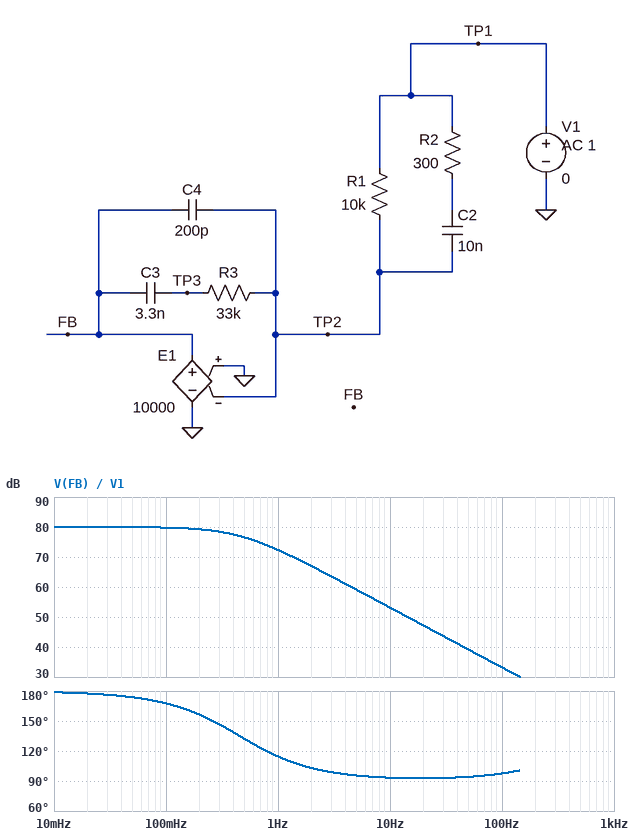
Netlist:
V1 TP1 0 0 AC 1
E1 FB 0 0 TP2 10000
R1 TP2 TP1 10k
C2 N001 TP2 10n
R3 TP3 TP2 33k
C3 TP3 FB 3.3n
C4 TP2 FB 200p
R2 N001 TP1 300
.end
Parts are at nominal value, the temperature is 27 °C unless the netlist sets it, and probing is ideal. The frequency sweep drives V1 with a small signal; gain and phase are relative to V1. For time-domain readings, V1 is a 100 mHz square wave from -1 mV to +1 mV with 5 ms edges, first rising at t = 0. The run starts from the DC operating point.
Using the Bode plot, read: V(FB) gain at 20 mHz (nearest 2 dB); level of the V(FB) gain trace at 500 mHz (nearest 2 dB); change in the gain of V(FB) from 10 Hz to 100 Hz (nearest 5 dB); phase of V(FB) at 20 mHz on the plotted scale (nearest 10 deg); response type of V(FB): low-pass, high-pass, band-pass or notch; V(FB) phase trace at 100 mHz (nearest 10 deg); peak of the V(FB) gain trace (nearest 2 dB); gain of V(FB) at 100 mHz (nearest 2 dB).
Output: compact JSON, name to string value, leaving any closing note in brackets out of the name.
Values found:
{"V(FB) gain at 20 mHz": "80 dB", "level of the V(FB) gain trace at 500 mHz": "76 dB", "change in the gain of V(FB) from 10 Hz to 100 Hz": "-20 dB", "phase of V(FB) at 20 mHz on the plotted scale": "180 deg", "response type of V(FB): low-pass, high-pass, band-pass or notch": "low-pass", "V(FB) phase trace at 100 mHz": "170 deg", "peak of the V(FB) gain trace": "80 dB", "gain of V(FB) at 100 mHz": "80 dB"}
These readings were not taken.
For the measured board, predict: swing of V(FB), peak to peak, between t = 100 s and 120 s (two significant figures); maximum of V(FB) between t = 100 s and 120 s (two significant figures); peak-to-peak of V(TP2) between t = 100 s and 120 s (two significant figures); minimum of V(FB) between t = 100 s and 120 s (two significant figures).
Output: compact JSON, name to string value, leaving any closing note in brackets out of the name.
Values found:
{"swing of V(FB), peak to peak, between t = 100 s and 120 s": "20 V", "maximum of V(FB) between t = 100 s and 120 s": "10 V", "peak-to-peak of V(TP2) between t = 100 s and 120 s": "2.0 mV", "minimum of V(FB) between t = 100 s and 120 s": "-10 V"}
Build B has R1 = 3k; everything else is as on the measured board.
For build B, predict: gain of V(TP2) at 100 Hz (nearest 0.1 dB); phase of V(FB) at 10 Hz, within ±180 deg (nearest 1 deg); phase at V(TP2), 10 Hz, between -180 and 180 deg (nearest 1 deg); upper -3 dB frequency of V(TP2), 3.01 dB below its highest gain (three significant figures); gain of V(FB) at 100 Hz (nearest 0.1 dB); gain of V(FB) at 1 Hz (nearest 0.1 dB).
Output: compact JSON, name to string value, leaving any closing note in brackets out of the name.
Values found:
{"gain of V(TP2) at 100 Hz": "-36.4 dB", "phase of V(FB) at 10 Hz, within ±180 deg": "99 deg", "phase at V(TP2), 10 Hz, between -180 and 180 deg": "-81 deg", "upper -3 dB frequency of V(TP2), 3.01 dB below its highest gain": "1.51 Hz", "gain of V(FB) at 100 Hz": "43.6 dB", "gain of V(FB) at 1 Hz": "78.4 dB"}
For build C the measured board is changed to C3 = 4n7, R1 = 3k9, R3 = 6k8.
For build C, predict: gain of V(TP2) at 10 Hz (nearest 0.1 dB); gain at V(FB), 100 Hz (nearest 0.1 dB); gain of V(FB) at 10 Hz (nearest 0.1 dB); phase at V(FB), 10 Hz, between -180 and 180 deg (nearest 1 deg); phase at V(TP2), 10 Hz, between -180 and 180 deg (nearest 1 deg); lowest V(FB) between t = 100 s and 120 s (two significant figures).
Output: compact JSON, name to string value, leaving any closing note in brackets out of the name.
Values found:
{"gain of V(TP2) at 10 Hz": "-21.6 dB", "gain at V(FB), 100 Hz": "38.4 dB", "gain of V(FB) at 10 Hz": "58.4 dB", "phase at V(FB), 10 Hz, between -180 and 180 deg": "95 deg", "phase at V(TP2), 10 Hz, between -180 and 180 deg": "-85 deg", "lowest V(FB) between t = 100 s and 120 s": "-10 V"}
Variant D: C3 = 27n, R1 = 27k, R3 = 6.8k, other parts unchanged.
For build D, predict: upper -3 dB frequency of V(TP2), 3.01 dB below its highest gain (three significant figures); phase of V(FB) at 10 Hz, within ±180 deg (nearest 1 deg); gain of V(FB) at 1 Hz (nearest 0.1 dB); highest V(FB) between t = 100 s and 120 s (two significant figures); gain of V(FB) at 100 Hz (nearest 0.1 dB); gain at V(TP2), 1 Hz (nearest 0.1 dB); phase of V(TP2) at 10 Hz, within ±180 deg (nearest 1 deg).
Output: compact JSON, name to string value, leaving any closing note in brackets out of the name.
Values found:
{"upper -3 dB frequency of V(TP2), 3.01 dB below its highest gain": "21.7 mHz", "phase of V(FB) at 10 Hz, within ±180 deg": "92 deg", "gain of V(FB) at 1 Hz": "46.7 dB", "highest V(FB) between t = 100 s and 120 s": "3.3 V", "gain of V(FB) at 100 Hz": "6.9 dB", "gain at V(TP2), 1 Hz": "-33.3 dB", "phase of V(TP2) at 10 Hz, within ±180 deg": "-88 deg"}
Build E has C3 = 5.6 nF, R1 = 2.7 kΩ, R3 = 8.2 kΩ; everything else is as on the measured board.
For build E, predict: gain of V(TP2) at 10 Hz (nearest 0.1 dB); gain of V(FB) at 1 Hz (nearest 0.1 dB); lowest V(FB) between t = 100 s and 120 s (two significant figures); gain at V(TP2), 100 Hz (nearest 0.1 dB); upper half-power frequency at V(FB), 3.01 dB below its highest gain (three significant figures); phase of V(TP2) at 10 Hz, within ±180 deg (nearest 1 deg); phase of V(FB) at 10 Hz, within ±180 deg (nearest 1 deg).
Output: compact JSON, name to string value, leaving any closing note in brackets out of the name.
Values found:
{"gain of V(TP2) at 10 Hz": "-19.9 dB", "gain of V(FB) at 1 Hz": "77.1 dB", "lowest V(FB) between t = 100 s and 120 s": "-10 V", "gain at V(TP2), 100 Hz": "-39.9 dB", "upper half-power frequency at V(FB), 3.01 dB below its highest gain": "1.02 Hz", "phase of V(TP2) at 10 Hz, within ±180 deg": "-84 deg", "phase of V(FB) at 10 Hz, within ±180 deg": "96 deg"}
